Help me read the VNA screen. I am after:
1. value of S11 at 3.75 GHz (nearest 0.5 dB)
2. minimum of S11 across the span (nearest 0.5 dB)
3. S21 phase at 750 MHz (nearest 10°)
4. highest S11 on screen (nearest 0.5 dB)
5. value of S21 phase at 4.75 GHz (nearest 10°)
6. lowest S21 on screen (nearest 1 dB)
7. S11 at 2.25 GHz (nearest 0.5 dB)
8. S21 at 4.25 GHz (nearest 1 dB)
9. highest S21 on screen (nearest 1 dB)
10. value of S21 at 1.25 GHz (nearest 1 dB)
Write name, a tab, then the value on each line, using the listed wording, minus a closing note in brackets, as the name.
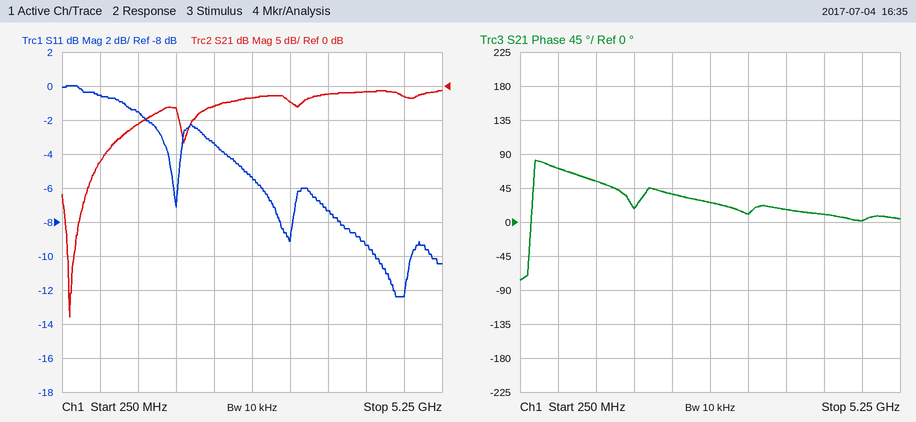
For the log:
value of S11 at 3.75 GHz	-7.5 dB
minimum of S11 across the span	-12.5 dB
S21 phase at 750 MHz	70°
highest S11 on screen	0.0 dB
value of S21 phase at 4.75 GHz	0°
lowest S21 on screen	-34 dB
S11 at 2.25 GHz	-3.5 dB
S21 at 4.25 GHz	-1 dB
highest S21 on screen	-1 dB
value of S21 at 1.25 GHz	-6 dB
